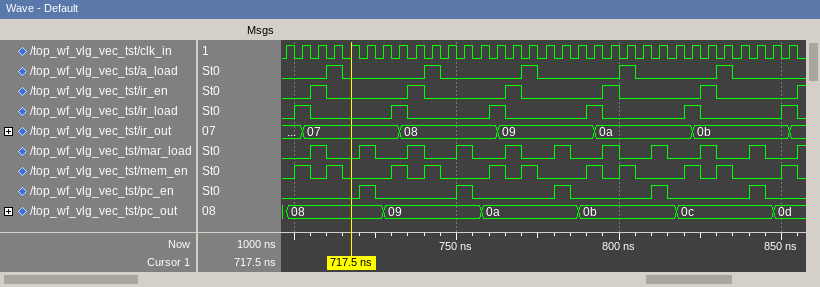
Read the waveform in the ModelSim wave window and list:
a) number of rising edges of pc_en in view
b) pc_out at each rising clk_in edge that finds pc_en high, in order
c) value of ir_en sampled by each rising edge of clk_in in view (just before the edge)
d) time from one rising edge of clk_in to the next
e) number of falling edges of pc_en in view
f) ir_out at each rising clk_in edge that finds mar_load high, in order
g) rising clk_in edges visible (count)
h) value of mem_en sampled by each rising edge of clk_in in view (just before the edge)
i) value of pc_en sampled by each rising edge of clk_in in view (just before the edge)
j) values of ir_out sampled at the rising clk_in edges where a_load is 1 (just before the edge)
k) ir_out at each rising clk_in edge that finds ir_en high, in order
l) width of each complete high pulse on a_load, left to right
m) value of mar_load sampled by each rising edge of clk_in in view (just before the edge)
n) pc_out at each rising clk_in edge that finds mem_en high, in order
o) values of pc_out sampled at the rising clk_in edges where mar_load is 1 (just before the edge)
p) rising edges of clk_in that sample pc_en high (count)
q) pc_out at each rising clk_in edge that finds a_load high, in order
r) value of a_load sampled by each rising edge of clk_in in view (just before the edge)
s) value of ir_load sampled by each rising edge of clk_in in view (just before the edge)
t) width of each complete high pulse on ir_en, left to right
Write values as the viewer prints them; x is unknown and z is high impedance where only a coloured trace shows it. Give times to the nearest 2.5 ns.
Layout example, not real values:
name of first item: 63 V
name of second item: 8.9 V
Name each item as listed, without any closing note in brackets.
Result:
number of rising edges of pc_en in view: 5
pc_out at each rising clk_in edge that finds pc_en high, in order: 08, 09, 0a, 0b, 0c
value of ir_en sampled by each rising edge of clk_in in view: 0 0 1 0 0 0 0 0 1 0 0 0 0 0 1 0 0 0 0 0 1 0 0 0 0 0 1 0 0 0 0 0
time from one rising edge of clk_in to the next: 5 ns
number of falling edges of pc_en in view: 5
ir_out at each rising clk_in edge that finds mar_load high, in order: 07, 07, 08, 08, 09, 09, 0a, 0a, 0b, 0b
rising clk_in edges visible: 32
value of mem_en sampled by each rising edge of clk_in in view: 0 1 0 1 0 0 0 1 0 1 0 0 0 1 0 1 0 0 0 1 0 1 0 0 0 1 0 1 0 0 0 1
value of pc_en sampled by each rising edge of clk_in in view: 0 0 0 0 0 1 0 0 0 0 0 1 0 0 0 0 0 1 0 0 0 0 0 1 0 0 0 0 0 1 0 0
values of ir_out sampled at the rising clk_in edges where a_load is 1: 07, 08, 09, 0a, 0b
ir_out at each rising clk_in edge that finds ir_en high, in order: 07, 08, 09, 0a, 0b
width of each complete high pulse on a_load, left to right: 5 ns, 5 ns, 5 ns, 5 ns, 5 ns
value of mar_load sampled by each rising edge of clk_in in view: 0 0 1 0 0 1 0 0 1 0 0 1 0 0 1 0 0 1 0 0 1 0 0 1 0 0 1 0 0 1 0 0
pc_out at each rising clk_in edge that finds mem_en high, in order: 08, 08, 09, 09, 0a, 0a, 0b, 0b, 0c, 0c, 0d
values of pc_out sampled at the rising clk_in edges where mar_load is 1: 08, 08, 09, 09, 0a, 0a, 0b, 0b, 0c, 0c
rising edges of clk_in that sample pc_en high: 5
pc_out at each rising clk_in edge that finds a_load high, in order: 08, 09, 0a, 0b, 0c
value of a_load sampled by each rising edge of clk_in in view: 0 0 0 1 0 0 0 0 0 1 0 0 0 0 0 1 0 0 0 0 0 1 0 0 0 0 0 1 0 0 0 0
value of ir_load sampled by each rising edge of clk_in in view: 0 1 0 0 0 0 0 1 0 0 0 0 0 1 0 0 0 0 0 1 0 0 0 0 0 1 0 0 0 0 0 1
width of each complete high pulse on ir_en, left to right: 5 ns, 5 ns, 5 ns, 5 ns, 5 ns
